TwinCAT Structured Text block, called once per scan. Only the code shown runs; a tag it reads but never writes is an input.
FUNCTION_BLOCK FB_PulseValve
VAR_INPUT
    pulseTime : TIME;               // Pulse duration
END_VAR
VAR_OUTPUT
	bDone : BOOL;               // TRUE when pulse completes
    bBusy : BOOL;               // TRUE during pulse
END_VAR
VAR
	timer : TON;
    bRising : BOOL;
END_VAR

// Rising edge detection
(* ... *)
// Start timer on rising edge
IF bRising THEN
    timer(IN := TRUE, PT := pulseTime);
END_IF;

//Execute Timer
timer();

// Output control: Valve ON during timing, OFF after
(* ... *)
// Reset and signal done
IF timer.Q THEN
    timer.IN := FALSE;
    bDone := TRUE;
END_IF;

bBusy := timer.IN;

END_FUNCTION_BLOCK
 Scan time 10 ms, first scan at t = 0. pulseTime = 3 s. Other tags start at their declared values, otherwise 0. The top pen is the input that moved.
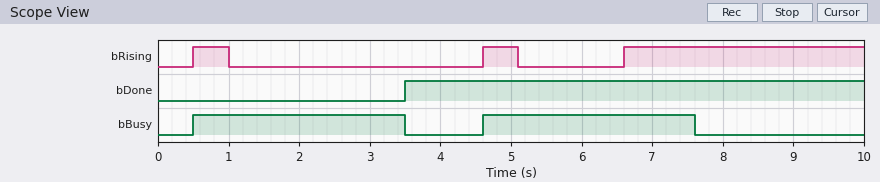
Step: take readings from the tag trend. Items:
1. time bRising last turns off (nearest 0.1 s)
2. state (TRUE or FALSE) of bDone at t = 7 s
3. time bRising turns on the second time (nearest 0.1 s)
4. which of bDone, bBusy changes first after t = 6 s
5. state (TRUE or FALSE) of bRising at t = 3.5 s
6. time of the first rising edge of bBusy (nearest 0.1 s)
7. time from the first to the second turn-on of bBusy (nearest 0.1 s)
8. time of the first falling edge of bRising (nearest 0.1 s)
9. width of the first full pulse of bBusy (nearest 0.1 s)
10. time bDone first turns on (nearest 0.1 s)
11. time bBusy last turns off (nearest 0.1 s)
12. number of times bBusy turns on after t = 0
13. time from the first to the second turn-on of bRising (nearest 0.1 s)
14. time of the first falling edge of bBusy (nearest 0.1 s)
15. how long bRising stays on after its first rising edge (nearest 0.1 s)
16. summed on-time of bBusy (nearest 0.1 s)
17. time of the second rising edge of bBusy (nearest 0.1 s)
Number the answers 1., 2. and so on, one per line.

1. 5.1 s
2. TRUE
3. 4.6 s
4. bBusy
5. FALSE
6. 0.5 s
7. 4.1 s
8. 1.0 s
9. 3.0 s
10. 3.5 s
11. 7.6 s
12. 2
13. 4.1 s
14. 3.5 s
15. 0.5 s
16. 6.0 s
17. 4.6 s
